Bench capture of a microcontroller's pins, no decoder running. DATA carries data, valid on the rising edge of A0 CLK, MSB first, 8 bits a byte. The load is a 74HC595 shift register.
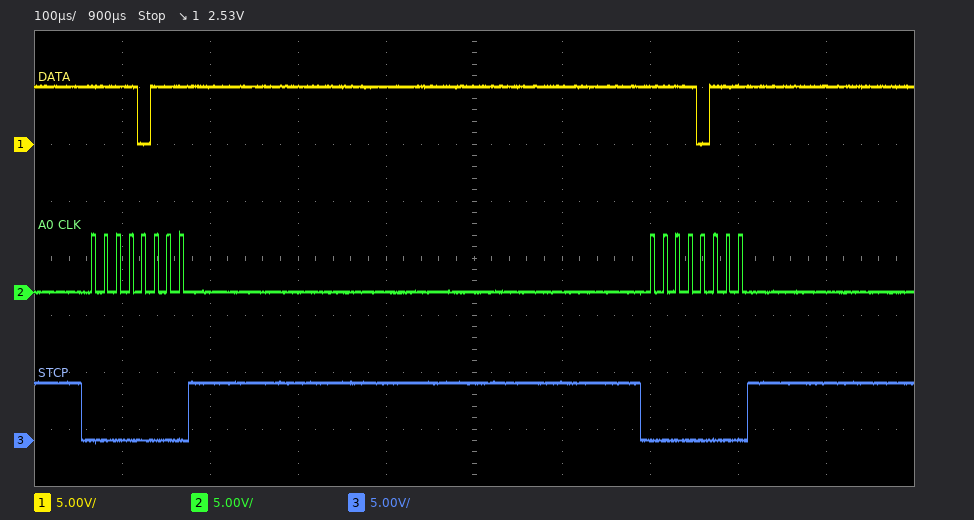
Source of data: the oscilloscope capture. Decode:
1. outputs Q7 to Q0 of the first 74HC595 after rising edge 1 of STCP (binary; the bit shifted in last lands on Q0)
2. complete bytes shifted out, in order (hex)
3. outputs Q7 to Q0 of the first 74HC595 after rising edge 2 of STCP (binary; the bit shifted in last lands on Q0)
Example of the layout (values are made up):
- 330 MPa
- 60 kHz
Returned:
- 11110111
- 0xF7 0xF7
- 11110111
